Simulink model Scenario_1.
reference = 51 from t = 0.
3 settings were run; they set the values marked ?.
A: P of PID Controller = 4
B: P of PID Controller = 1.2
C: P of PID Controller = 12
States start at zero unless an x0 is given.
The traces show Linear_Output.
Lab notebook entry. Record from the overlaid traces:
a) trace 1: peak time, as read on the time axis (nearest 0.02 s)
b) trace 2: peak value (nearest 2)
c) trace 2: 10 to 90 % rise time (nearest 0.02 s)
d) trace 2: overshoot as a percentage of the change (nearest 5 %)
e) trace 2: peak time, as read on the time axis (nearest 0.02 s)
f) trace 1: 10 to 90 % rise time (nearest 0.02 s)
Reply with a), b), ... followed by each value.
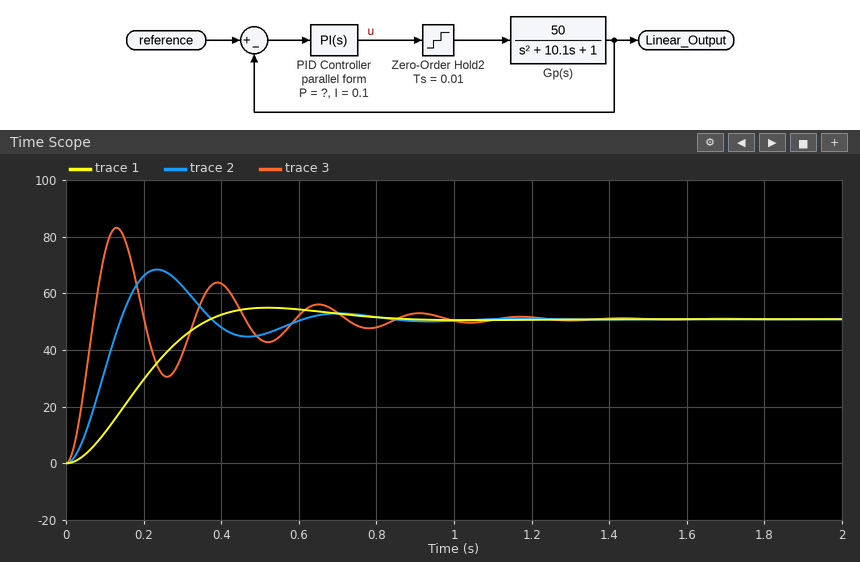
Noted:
a) 0.52 s
b) 68
c) 0.10 s
d) 35 %
e) 0.24 s
f) 0.24 s
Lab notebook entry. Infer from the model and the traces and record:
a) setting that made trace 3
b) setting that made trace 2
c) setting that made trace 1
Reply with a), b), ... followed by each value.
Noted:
a) C
b) A
c) B
